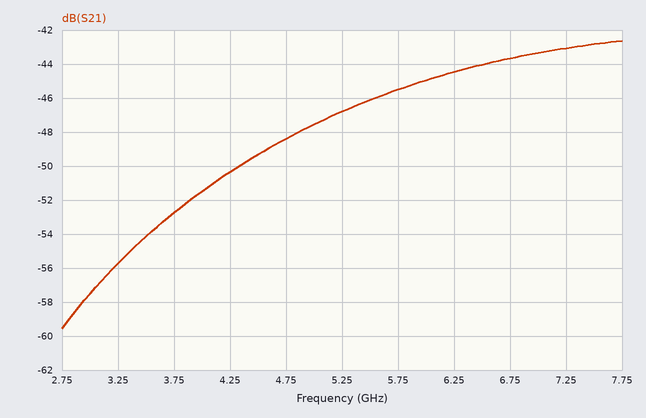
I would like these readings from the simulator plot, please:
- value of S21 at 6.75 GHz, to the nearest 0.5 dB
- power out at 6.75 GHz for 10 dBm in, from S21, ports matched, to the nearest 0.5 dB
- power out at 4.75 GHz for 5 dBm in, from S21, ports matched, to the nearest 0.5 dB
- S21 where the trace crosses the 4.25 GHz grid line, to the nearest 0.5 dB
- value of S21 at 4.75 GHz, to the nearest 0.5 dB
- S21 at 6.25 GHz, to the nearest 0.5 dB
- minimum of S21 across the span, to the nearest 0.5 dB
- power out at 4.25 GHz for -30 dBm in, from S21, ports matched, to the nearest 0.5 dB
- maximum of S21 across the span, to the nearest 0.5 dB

-43.5 dB
-33.5 dBm
-43.5 dBm
-50.5 dB
-48.5 dB
-44.5 dB
-59.5 dB
-80.5 dBm
-42.5 dB
